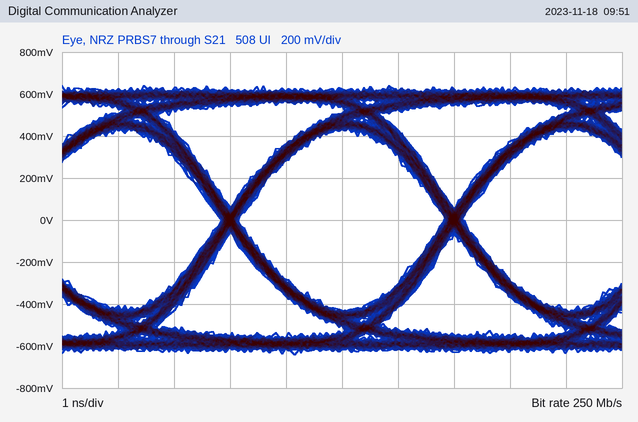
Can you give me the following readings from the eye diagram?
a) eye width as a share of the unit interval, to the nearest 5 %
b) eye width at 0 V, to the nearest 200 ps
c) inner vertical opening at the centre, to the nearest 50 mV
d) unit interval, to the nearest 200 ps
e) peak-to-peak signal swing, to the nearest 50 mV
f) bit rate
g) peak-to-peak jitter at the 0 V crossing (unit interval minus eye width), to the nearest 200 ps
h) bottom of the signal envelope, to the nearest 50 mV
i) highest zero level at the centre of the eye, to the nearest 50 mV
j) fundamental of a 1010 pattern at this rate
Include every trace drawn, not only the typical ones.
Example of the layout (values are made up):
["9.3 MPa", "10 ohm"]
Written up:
["90 %", "3.6 ns", "850 mV", "4.0 ns", "1.30 V", "250 Mb/s", "400 ps", "-650 mV", "-450 mV", "125 MHz"]
